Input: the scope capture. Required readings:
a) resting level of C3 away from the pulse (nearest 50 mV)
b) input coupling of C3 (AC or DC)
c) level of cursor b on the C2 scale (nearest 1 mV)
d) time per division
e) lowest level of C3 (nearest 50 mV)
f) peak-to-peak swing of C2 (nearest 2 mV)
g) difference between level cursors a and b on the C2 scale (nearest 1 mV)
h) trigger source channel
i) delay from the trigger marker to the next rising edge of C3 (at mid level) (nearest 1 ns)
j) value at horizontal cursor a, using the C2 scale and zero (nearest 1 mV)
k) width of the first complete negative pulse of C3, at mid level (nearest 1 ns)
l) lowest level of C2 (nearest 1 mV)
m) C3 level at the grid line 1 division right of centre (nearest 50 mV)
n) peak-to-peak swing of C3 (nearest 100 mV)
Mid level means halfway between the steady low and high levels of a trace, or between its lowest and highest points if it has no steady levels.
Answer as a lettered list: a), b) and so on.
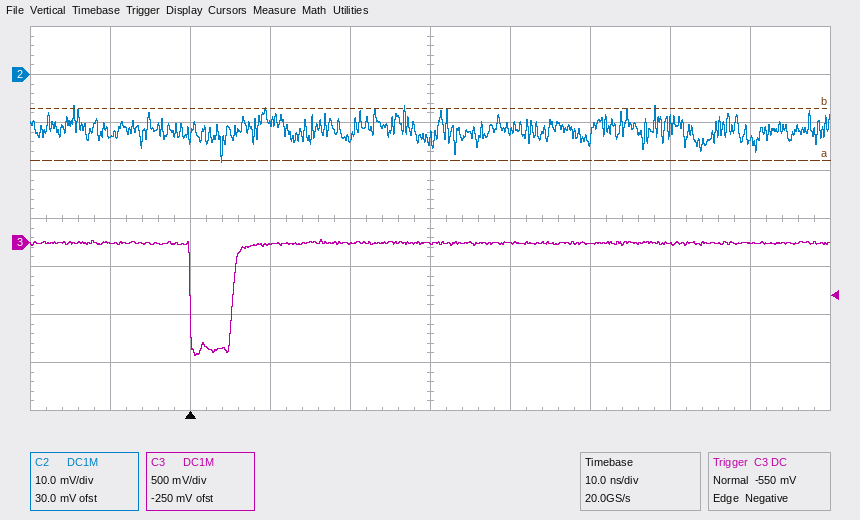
a) 0 mV
b) DC
c) -7 mV
d) 10 ns
e) -1.20 V
f) 12 mV
g) 11 mV
h) C3
i) 5 ns
j) -18 mV
k) 5 ns
l) -18 mV
m) 0 mV
n) 1.20 V
